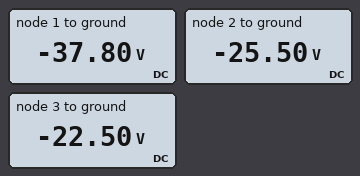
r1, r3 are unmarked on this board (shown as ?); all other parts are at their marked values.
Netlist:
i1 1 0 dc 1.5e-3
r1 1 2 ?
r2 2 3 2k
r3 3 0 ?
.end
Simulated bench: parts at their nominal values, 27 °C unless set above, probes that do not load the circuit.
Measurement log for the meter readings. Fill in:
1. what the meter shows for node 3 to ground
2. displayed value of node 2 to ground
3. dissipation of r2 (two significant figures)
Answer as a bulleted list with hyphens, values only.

- -22.50 V
- -25.50 V
- 4.5 mW
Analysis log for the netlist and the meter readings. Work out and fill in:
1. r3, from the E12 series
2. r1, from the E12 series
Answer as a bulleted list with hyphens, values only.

- 15 kΩ
- 8.2 kΩ
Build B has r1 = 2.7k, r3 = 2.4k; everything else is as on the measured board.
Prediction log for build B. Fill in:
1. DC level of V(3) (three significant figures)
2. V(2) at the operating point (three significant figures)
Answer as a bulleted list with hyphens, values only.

- -3.60 V
- -6.60 V
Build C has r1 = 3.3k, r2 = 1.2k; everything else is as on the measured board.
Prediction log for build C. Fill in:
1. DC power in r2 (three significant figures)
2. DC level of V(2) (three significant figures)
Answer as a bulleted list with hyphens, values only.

- 2.70 mW
- -24.3 V
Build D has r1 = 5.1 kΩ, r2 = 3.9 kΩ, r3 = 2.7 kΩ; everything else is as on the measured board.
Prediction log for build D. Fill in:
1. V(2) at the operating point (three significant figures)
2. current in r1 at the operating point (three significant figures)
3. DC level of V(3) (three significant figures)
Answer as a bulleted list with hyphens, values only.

- -9.90 V
- 1.50 mA
- -4.05 V
